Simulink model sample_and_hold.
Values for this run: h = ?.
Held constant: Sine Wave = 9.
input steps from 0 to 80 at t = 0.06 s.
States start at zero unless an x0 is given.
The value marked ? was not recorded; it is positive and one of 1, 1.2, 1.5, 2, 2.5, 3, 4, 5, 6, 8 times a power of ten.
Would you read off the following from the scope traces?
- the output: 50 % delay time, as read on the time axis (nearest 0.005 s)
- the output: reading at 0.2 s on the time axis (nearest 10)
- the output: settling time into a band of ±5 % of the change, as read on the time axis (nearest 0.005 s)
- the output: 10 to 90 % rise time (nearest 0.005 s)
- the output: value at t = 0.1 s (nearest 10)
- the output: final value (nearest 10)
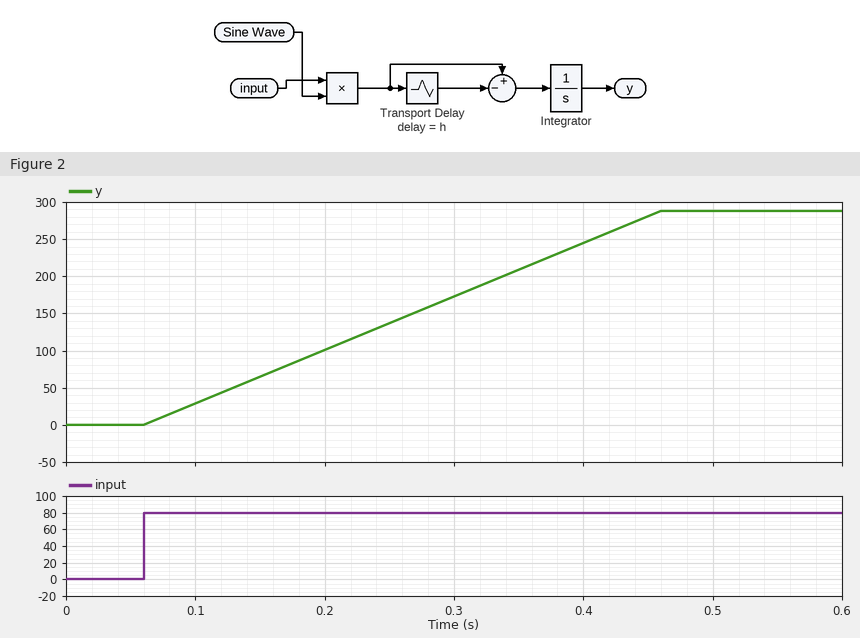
0.260 s
100
0.440 s
0.320 s
30
290
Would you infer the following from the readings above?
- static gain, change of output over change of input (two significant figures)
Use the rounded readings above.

3.6
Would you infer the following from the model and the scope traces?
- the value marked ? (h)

0.4
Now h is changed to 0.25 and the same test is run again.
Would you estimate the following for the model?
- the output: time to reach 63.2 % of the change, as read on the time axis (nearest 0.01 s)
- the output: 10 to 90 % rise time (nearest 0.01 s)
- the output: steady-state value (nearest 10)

0.22 s
0.20 s
180
